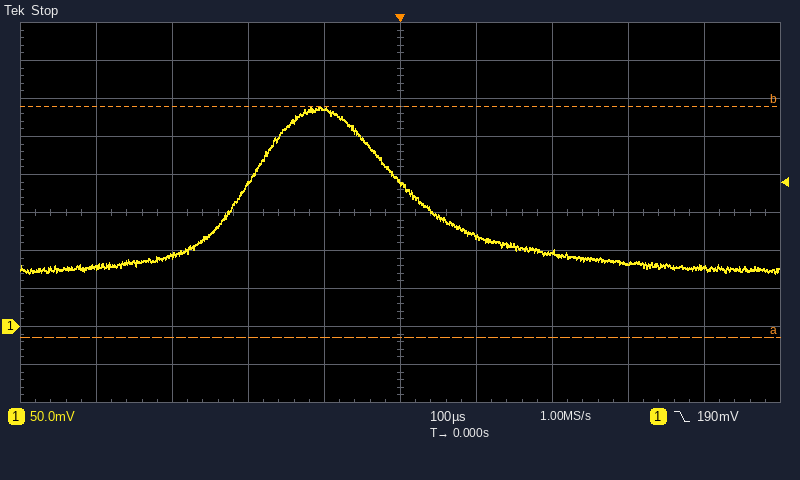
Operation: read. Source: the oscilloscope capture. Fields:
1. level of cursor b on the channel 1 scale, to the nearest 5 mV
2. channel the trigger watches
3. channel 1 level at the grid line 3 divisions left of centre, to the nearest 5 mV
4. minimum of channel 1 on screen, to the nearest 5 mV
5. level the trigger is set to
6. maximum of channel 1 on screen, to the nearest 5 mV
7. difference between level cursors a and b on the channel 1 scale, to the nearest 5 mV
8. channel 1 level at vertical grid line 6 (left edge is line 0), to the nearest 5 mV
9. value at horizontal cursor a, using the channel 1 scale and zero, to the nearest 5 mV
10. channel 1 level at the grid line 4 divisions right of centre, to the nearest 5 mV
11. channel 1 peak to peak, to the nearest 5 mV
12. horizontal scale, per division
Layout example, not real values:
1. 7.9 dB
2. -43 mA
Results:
1. 290 mV
2. channel 1
3. 95 mV
4. 70 mV
5. 190 mV
6. 290 mV
7. 305 mV
8. 120 mV
9. -15 mV
10. 75 mV
11. 220 mV
12. 100 µs
